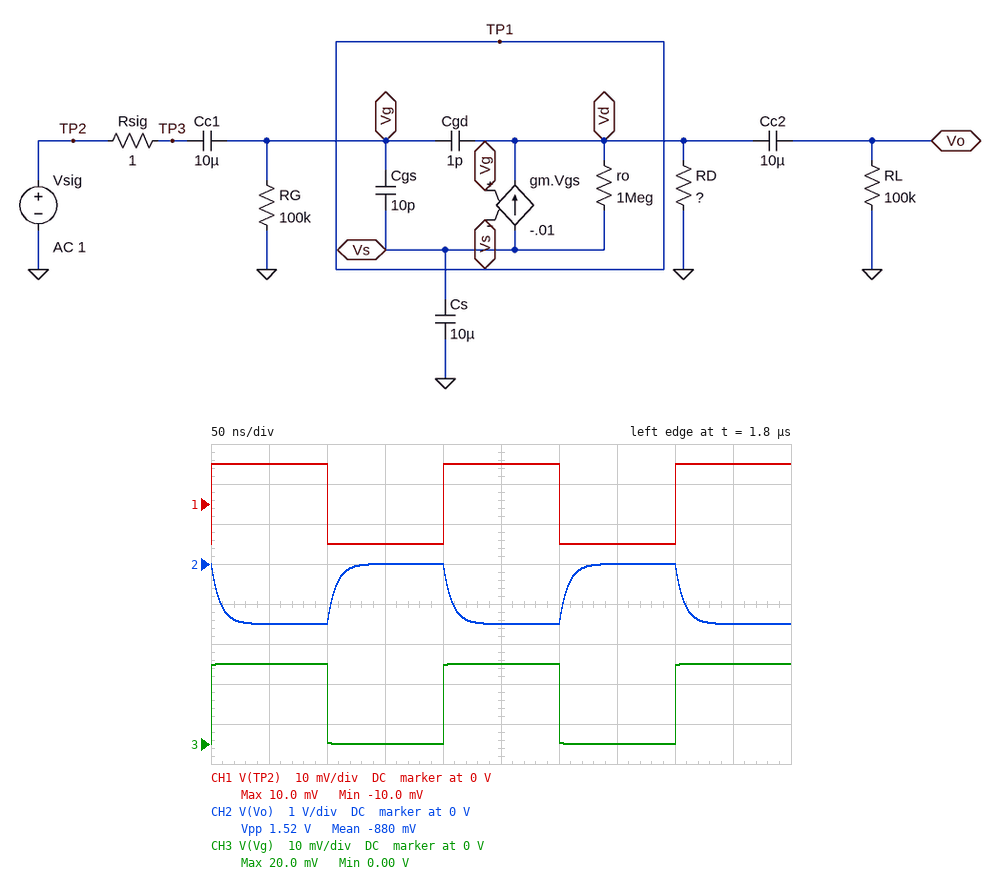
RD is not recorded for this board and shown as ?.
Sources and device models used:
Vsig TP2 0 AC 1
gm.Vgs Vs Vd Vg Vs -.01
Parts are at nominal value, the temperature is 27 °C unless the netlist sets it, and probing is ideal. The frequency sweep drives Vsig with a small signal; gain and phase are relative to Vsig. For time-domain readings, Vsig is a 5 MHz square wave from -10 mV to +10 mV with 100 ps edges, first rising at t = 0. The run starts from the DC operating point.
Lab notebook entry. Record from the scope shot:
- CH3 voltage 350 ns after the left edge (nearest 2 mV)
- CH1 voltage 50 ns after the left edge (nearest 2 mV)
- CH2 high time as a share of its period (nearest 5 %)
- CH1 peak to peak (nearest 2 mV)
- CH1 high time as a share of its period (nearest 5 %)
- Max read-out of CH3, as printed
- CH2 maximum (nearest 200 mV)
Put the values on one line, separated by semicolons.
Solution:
0 V; 10 mV; 50 %; 20 mV; 50 %; 20.0 mV; 0 V
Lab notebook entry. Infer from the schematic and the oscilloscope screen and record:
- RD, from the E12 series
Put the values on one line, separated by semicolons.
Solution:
8.2 kΩ
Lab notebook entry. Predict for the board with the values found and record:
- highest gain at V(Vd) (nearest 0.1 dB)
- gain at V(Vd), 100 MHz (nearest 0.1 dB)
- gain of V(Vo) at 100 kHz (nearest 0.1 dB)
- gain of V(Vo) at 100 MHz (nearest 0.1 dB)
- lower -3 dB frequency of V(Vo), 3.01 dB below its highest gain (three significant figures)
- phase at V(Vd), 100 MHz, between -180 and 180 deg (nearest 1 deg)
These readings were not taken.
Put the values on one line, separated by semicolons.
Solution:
37.5 dB; 23.8 dB; 37.5 dB; 23.8 dB; 158 Hz; 98 deg
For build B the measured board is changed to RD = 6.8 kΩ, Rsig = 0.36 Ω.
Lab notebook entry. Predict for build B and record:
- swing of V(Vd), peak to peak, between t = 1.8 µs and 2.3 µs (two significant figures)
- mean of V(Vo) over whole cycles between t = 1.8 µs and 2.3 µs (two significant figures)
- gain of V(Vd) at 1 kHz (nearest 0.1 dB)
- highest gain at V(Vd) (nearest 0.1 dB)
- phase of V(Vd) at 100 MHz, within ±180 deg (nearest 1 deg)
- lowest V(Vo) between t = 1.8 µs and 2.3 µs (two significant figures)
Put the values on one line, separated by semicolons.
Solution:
1.3 V; -630 mV; 35.9 dB; 36.0 dB; 100 deg; -1.3 V
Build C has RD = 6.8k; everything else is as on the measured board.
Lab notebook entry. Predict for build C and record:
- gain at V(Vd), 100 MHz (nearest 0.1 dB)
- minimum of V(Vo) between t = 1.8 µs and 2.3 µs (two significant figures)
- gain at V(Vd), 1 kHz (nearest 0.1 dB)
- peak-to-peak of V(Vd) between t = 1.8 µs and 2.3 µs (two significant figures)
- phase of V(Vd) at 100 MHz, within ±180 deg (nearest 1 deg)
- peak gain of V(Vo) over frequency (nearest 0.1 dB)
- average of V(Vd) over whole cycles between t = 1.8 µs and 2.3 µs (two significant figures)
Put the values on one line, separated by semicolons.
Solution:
23.7 dB; -1.3 V; 35.9 dB; 1.3 V; 100 deg; 36.0 dB; -630 mV
